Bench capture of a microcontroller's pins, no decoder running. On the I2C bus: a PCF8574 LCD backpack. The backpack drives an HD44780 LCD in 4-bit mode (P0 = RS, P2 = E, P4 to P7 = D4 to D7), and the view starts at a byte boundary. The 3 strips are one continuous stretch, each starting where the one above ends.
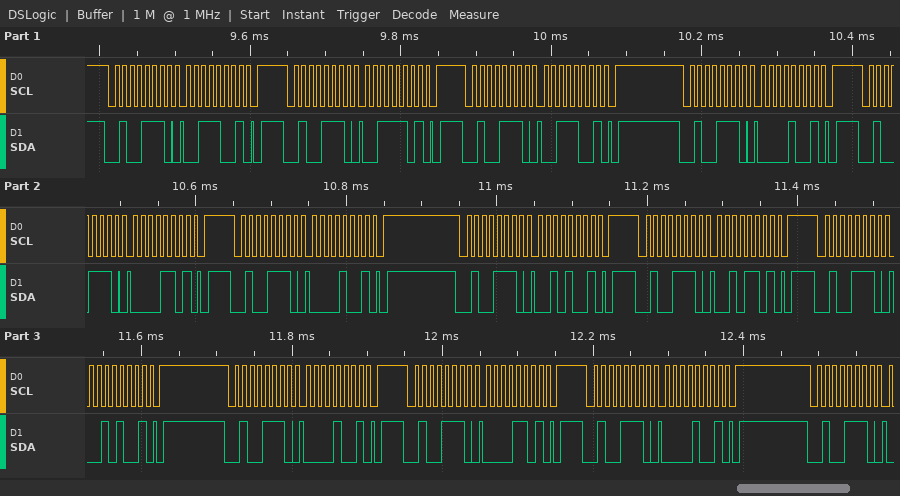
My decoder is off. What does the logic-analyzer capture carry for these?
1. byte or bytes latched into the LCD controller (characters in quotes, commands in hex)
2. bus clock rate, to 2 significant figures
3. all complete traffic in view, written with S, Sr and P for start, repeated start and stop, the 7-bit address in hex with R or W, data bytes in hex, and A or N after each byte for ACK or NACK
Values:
'0' ' '
100 kHz
S 27W A 39 A P S 27W A 3D A P S 27W A 39 A P S 27W A 09 A P S 27W A 0D A P S 27W A 09 A P S 27W A 29 A P S 27W A 2D A P S 27W A 29 A P S 27W A 09 A P S 27W A 0D A P S 27W A 09 A P S 27W A
